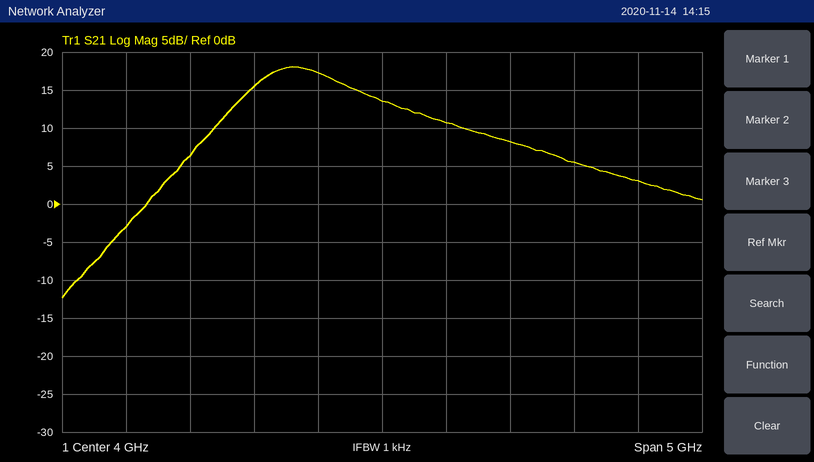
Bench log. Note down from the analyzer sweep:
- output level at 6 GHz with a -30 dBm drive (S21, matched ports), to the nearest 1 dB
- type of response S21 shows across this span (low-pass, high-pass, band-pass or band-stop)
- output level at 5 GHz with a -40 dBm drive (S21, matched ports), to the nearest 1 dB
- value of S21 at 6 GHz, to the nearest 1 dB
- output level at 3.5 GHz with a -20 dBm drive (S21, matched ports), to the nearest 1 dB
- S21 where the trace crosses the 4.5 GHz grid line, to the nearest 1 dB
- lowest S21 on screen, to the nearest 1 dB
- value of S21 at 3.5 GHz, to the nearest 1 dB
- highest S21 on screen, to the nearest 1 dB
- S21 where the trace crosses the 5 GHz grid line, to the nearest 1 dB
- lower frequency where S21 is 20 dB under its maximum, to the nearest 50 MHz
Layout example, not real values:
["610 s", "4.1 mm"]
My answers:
["-27 dBm", "band-pass", "-32 dBm", "3 dB", "-3 dBm", "11 dB", "-12 dB", "17 dB", "18 dB", "8 dB", "2.05 GHz"]
